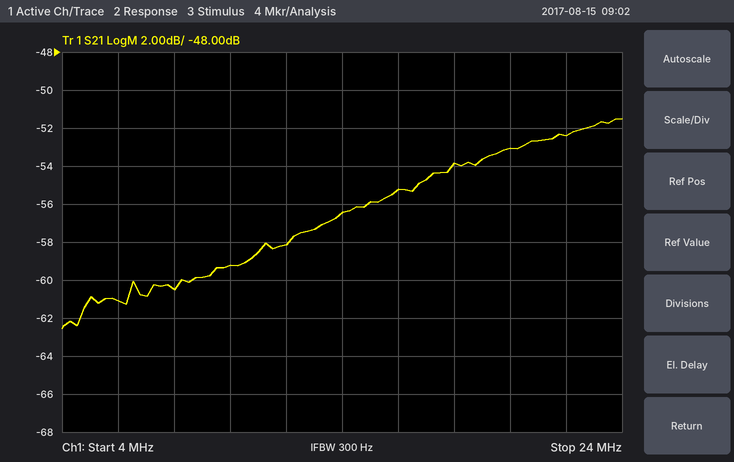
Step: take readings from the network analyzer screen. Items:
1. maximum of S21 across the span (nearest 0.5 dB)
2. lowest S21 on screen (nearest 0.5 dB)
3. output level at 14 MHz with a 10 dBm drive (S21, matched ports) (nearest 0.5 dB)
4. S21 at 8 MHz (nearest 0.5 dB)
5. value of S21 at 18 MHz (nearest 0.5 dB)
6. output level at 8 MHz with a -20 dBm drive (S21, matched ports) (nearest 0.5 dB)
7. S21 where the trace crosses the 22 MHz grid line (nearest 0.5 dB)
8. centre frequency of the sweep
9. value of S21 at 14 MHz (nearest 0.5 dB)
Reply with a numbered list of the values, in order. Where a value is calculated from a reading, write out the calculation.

1. -51.5 dB
2. -62.5 dB
3. 10 dBm + (-56.5 dB) = -46.5 dBm
4. -60.5 dB
5. -54.0 dB
6. -20 dBm + (-60.5 dB) = -80.5 dBm
7. -52.5 dB
8. 14 MHz
9. -56.5 dB
